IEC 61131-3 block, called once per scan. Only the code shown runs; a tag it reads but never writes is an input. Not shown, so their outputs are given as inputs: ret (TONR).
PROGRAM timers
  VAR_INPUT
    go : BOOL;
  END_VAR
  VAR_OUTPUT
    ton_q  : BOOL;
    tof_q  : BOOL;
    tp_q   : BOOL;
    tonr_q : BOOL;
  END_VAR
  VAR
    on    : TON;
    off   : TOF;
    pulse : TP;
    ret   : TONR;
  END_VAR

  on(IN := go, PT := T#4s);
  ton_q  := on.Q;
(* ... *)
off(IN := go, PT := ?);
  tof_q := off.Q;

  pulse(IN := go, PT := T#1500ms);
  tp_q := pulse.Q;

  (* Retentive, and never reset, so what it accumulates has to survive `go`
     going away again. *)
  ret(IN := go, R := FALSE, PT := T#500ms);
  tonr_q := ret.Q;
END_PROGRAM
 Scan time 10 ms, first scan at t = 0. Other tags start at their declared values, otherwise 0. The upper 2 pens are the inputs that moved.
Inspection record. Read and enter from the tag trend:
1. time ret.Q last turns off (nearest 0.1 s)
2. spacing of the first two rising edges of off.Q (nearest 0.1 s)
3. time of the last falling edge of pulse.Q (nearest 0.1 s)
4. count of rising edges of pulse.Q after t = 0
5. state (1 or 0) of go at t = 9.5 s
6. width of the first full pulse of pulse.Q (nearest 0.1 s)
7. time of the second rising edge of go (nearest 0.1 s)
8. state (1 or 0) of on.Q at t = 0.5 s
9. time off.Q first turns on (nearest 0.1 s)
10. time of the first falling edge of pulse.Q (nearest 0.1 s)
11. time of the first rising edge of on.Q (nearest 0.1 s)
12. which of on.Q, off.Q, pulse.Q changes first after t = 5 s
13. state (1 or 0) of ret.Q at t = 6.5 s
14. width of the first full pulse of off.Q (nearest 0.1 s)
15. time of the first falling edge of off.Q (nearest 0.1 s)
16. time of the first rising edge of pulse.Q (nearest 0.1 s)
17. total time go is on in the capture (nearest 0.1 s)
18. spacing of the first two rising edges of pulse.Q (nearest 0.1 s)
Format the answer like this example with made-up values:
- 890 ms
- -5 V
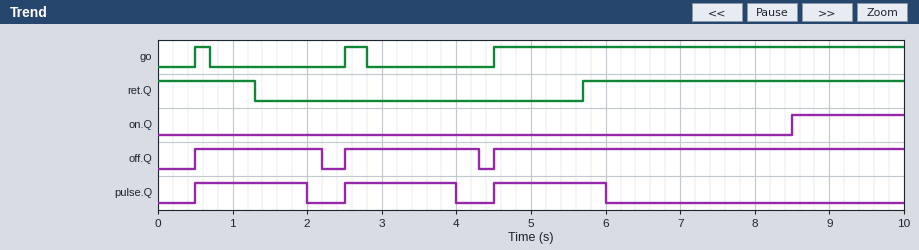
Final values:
- 1.3 s
- 2.0 s
- 6.0 s
- 3
- 1
- 1.5 s
- 2.5 s
- 0
- 0.5 s
- 2.0 s
- 8.5 s
- pulse.Q
- 1
- 1.7 s
- 2.2 s
- 0.5 s
- 6.0 s
- 2.0 s
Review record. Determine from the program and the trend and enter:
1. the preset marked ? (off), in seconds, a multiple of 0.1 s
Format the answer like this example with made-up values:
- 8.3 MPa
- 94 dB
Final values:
- 1.5 s
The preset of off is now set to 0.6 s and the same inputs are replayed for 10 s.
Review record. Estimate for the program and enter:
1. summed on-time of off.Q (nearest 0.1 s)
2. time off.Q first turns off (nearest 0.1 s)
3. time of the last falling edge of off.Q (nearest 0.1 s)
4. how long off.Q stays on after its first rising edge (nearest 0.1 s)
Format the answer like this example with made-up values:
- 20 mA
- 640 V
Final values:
- 7.2 s
- 1.3 s
- 3.4 s
- 0.8 s
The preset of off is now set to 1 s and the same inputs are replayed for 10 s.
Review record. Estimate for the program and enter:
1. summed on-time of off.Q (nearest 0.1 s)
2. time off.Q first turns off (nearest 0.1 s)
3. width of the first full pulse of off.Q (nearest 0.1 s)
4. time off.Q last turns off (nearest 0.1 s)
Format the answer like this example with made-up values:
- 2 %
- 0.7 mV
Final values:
- 8.0 s
- 1.7 s
- 1.2 s
- 3.8 s
